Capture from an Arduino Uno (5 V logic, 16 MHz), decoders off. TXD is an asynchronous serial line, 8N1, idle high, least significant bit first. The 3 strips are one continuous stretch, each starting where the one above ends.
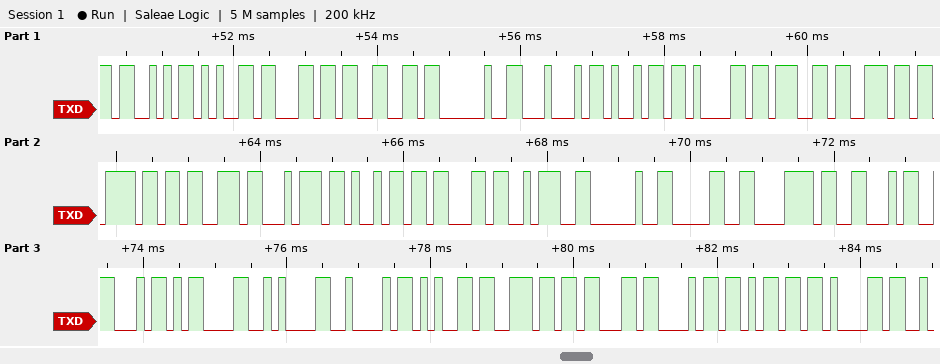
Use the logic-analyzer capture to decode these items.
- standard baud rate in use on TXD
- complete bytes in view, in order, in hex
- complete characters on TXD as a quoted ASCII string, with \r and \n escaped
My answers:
9600 baud
53 65 6C 66 20 44 69 61 67 6E 6F 73 74 69 63 3A 20 30 78 46 46 0D 0A 42 65 6E 63 68 6D 61
"Self Diagnostic: 0xFF\r\nBenchma"
